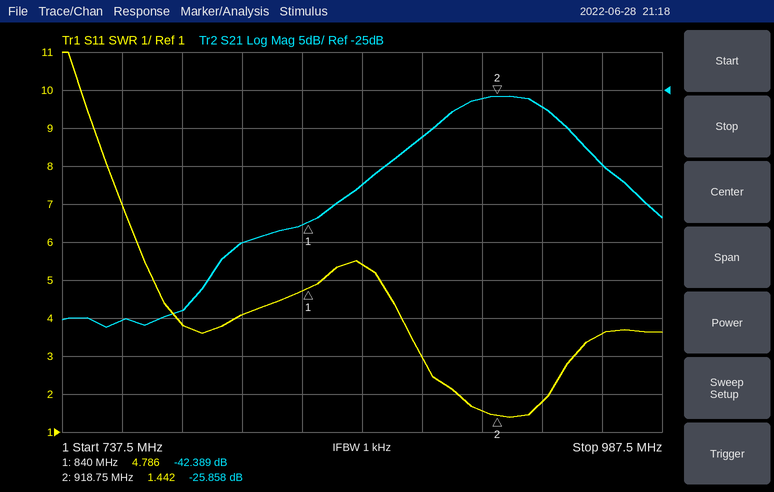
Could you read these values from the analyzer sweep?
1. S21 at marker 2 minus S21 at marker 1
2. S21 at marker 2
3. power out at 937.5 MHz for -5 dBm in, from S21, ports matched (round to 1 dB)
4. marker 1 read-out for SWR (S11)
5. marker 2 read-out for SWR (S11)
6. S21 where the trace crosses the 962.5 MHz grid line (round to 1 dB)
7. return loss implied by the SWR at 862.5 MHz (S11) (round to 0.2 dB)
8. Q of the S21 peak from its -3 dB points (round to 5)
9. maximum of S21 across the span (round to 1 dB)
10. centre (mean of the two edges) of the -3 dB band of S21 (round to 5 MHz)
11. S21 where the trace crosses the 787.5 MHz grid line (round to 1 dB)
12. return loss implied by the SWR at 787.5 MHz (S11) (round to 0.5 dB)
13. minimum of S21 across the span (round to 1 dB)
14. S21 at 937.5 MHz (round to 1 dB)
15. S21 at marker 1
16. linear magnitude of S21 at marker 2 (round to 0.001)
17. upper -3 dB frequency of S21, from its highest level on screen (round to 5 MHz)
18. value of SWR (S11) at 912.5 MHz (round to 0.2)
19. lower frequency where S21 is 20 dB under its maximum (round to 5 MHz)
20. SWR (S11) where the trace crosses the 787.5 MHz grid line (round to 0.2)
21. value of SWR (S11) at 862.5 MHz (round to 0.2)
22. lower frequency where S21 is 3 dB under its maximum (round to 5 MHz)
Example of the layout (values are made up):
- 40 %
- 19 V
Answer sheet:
- 16.531 dB
- -25.858 dB
- -32 dBm
- 4.786
- 1.442
- -35 dB
- 3.2 dB
- 20
- -26 dB
- 920 MHz
- -54 dB
- 4.5 dB
- -56 dB
- -27 dB
- -42.389 dB
- 0.051
- 945 MHz
- 1.6
- 810 MHz
- 3.8
- 5.4
- 895 MHz
